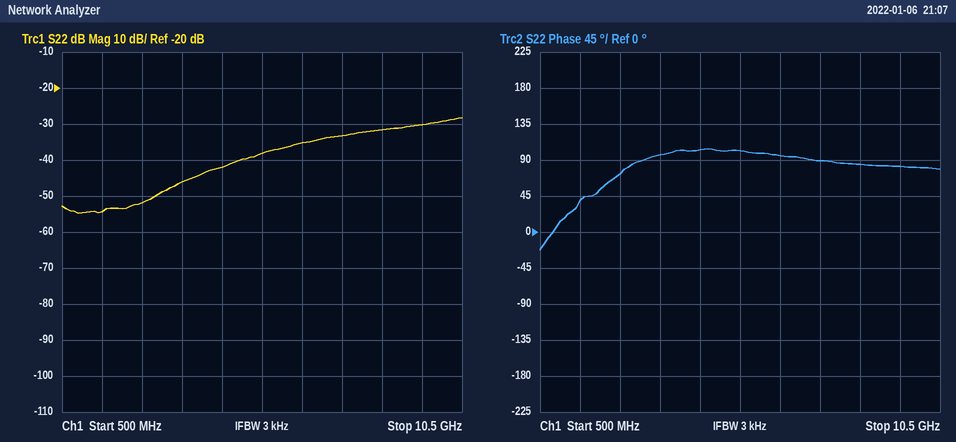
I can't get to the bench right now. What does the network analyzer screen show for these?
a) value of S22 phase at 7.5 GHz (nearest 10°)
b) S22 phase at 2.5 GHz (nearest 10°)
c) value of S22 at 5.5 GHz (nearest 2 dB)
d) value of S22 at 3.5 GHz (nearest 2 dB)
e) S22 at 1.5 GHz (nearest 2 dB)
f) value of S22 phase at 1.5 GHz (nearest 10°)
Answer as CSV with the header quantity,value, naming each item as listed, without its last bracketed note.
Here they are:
quantity,value
value of S22 phase at 7.5 GHz,90°
S22 phase at 2.5 GHz,70°
value of S22 at 5.5 GHz,-38 dB
value of S22 at 3.5 GHz,-46 dB
S22 at 1.5 GHz,-54 dB
value of S22 phase at 1.5 GHz,40°
